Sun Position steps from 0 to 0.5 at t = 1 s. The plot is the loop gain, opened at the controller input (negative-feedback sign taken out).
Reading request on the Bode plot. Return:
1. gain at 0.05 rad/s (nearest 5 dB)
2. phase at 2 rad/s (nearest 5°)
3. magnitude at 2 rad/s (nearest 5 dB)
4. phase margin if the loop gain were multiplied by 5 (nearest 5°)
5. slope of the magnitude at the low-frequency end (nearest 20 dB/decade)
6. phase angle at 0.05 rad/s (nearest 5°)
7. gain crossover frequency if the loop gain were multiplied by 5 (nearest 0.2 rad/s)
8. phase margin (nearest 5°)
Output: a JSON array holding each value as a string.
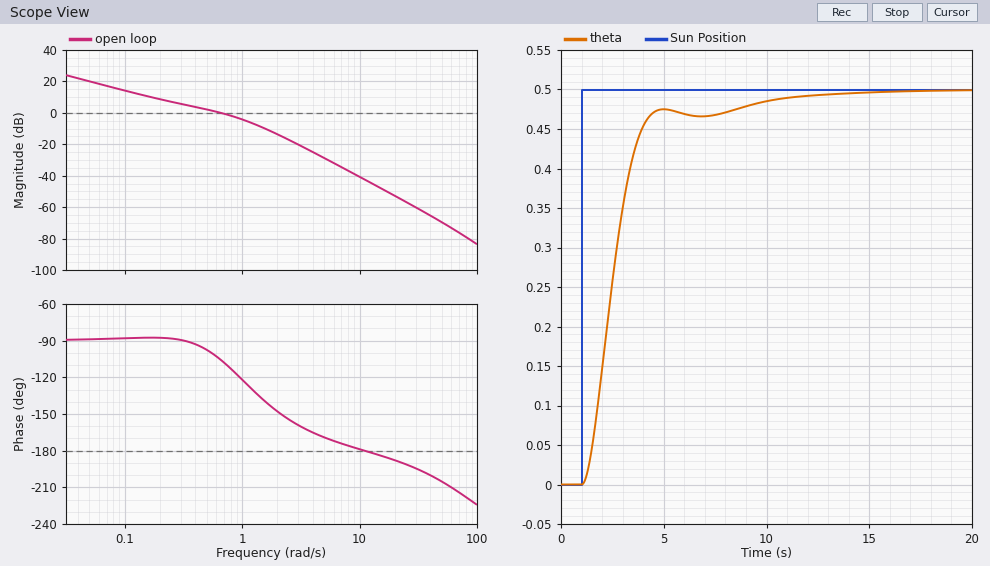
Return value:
["20 dB", "-150°", "-15 dB", "30°", "-20 dB/decade", "-90°", "2.0 rad/s", "75°"]
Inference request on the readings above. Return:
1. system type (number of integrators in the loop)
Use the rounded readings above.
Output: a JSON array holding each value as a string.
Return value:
["1"]
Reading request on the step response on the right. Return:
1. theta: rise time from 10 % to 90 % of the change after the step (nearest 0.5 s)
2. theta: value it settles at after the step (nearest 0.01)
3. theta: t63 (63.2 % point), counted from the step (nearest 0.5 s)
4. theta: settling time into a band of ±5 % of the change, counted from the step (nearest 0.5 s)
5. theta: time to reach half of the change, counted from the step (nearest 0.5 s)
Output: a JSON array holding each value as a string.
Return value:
["2.5 s", "0.50", "2.0 s", "7.5 s", "1.5 s"]
